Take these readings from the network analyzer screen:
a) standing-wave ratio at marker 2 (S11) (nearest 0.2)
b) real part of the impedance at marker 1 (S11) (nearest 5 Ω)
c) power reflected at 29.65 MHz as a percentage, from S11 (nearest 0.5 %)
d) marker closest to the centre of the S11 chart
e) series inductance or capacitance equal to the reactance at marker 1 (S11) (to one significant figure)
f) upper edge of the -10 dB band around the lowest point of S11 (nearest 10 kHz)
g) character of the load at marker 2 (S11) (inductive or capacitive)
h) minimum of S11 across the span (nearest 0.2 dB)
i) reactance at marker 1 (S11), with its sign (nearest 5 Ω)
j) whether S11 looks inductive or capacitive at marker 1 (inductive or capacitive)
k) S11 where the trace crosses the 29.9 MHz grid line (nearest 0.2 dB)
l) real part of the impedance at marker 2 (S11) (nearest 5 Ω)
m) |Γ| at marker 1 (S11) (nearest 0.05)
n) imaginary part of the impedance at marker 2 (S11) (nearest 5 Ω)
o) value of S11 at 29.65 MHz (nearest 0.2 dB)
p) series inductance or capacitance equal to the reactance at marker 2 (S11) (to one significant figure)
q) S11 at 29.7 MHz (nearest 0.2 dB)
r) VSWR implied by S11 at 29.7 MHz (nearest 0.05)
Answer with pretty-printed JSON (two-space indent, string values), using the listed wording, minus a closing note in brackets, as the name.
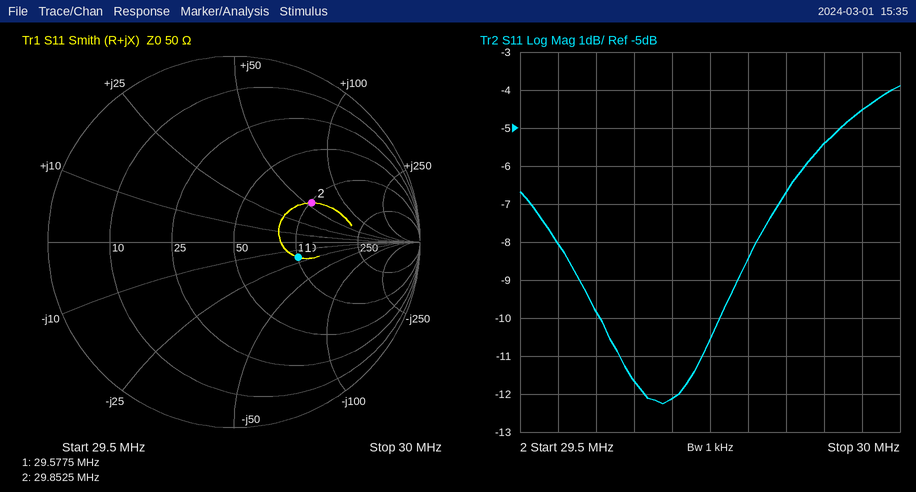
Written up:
{
  "standing-wave ratio at marker 2 (S11)": "2.8",
  "real part of the impedance at marker 1 (S11)": "100 Ω",
  "power reflected at 29.65 MHz as a percentage, from S11": "7.0 %",
  "marker closest to the centre of the S11 chart": "marker 1",
  "series inductance or capacitance equal to the reactance at marker 1 (S11)": "300 pF",
  "upper edge of the -10 dB band around the lowest point of S11": "29.76 MHz",
  "character of the load at marker 2 (S11)": "inductive",
  "minimum of S11 across the span": "-12.2 dB",
  "reactance at marker 1 (S11), with its sign": "-20 Ω",
  "whether S11 looks inductive or capacitive at marker 1": "capacitive",
  "S11 where the trace crosses the 29.9 MHz grid line": "-5.4 dB",
  "real part of the impedance at marker 2 (S11)": "100 Ω",
  "|Γ| at marker 1 (S11)": "0.35",
  "imaginary part of the impedance at marker 2 (S11)": "+55 Ω",
  "value of S11 at 29.65 MHz": "-11.6 dB",
  "series inductance or capacitance equal to the reactance at marker 2 (S11)": "300 nH",
  "S11 at 29.7 MHz": "-12.2 dB",
  "VSWR implied by S11 at 29.7 MHz": "1.65"
}
